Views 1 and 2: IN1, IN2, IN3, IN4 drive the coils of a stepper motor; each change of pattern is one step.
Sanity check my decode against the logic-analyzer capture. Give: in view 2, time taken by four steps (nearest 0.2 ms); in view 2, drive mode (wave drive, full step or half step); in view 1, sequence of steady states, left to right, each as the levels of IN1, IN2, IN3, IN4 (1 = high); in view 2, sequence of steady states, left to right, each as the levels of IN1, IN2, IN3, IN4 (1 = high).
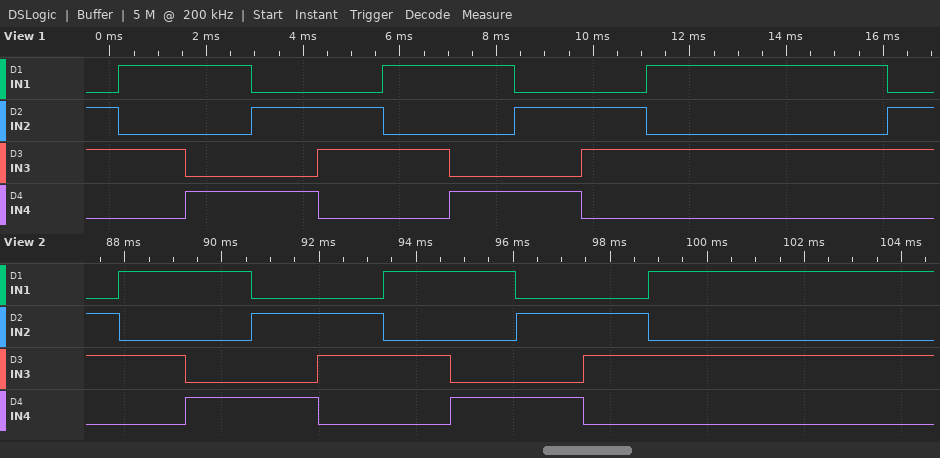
5.4 ms
full step
0110 1010 1001 0101 0110 1010 1001 0101 0110 1010 0110
0110 1010 1001 0101 0110 1010 1001 0101 0110 1010
